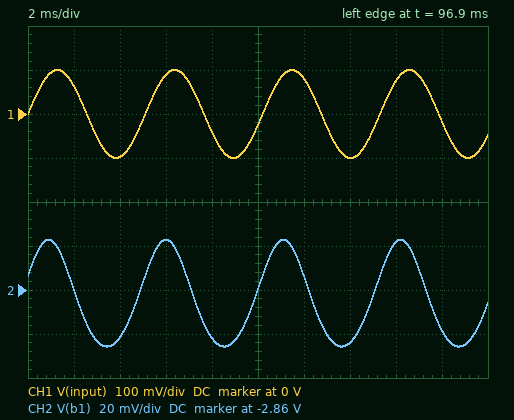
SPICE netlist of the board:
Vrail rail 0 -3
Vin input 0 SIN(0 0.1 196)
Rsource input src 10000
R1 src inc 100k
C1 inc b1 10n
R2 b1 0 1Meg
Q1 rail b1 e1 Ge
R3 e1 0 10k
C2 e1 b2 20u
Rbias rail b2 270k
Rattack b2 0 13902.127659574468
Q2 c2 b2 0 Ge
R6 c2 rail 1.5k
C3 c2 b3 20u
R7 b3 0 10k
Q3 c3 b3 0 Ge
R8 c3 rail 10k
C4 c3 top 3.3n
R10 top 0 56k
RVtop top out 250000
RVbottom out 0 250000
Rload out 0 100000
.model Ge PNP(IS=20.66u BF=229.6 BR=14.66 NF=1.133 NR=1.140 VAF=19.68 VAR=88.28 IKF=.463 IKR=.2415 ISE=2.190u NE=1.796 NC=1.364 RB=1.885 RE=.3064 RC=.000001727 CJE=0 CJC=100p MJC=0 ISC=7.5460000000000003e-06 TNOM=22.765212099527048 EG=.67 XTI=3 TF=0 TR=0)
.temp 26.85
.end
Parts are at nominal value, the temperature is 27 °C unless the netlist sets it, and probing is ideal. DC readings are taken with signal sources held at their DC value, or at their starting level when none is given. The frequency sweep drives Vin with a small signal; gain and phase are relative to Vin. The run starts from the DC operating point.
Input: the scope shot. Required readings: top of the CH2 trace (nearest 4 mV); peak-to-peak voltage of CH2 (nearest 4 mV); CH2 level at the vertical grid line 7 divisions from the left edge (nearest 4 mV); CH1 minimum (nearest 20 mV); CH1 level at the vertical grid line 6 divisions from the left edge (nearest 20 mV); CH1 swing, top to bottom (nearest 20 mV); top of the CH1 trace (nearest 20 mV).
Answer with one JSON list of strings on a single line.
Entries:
["-2.836 V", "48 mV", "-2.884 V", "-100 mV", "80 mV", "200 mV", "100 mV"]
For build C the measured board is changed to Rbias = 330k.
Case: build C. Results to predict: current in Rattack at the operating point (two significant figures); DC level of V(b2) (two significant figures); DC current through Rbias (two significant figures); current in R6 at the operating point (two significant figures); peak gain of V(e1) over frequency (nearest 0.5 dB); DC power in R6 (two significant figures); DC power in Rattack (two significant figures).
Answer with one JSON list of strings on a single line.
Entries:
["5.9 µA", "-82 mV", "8.8 µA", "560 µA", "-11.5 dB", "480 µW", "480 nW"]
